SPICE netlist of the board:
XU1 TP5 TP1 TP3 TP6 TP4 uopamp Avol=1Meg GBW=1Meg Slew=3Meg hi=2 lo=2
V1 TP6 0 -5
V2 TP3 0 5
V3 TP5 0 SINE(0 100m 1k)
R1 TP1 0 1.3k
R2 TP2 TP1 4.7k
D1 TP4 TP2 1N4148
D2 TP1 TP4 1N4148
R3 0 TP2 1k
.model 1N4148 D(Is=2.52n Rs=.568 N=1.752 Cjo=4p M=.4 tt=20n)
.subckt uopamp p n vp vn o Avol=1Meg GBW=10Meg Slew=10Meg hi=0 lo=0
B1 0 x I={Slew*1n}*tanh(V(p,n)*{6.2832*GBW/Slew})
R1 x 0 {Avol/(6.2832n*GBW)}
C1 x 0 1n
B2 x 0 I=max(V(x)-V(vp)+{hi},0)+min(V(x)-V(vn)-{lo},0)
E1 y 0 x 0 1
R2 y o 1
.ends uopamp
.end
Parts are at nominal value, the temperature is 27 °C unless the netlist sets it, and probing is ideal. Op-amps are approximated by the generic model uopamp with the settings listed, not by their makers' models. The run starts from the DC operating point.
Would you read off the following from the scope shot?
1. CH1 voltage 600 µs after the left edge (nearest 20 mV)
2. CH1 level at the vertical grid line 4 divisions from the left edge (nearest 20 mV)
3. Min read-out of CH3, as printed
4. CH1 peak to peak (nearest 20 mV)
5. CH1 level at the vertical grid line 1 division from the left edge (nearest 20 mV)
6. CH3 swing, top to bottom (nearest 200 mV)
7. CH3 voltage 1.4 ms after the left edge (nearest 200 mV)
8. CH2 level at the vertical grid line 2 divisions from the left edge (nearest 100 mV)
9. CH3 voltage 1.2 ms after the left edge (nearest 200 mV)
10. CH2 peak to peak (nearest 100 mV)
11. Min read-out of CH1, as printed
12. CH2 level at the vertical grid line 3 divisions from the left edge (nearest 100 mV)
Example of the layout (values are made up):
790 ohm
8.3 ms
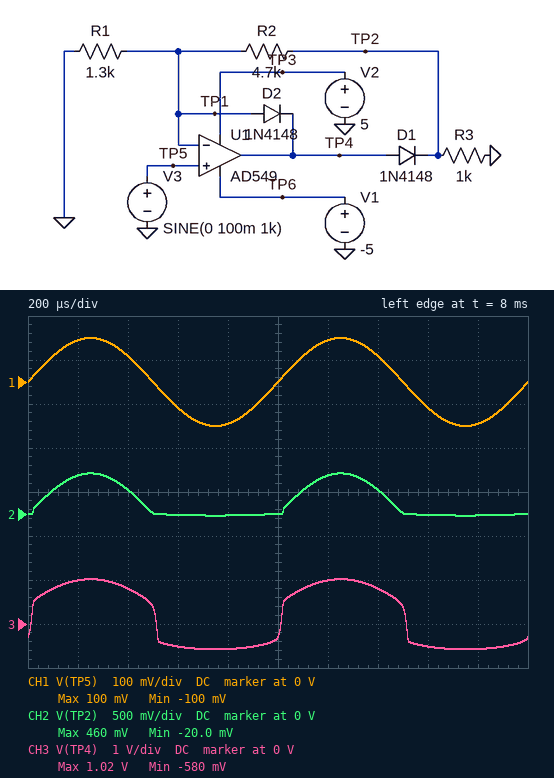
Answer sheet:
-60 mV
-100 mV
-580 mV
200 mV
100 mV
1.6 V
800 mV
300 mV
1.0 V
500 mV
-100 mV
0 V
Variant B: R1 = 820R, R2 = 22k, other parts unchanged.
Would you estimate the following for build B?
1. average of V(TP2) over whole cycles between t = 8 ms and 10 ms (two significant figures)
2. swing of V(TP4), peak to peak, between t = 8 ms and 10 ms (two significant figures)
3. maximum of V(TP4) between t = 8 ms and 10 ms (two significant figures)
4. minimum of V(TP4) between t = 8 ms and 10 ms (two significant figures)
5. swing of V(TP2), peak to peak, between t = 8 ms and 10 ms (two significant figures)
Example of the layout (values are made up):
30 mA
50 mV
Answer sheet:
830 mV
3.6 V
3.0 V
-590 mV
2.4 V
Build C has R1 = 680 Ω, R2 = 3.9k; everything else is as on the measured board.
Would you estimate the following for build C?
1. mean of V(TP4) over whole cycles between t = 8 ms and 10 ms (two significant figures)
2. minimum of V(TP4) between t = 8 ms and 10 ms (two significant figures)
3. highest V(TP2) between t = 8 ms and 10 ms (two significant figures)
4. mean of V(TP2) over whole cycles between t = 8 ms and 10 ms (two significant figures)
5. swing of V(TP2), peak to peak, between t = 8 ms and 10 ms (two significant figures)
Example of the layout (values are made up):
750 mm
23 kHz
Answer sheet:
220 mV
-600 mV
670 mV
210 mV
690 mV
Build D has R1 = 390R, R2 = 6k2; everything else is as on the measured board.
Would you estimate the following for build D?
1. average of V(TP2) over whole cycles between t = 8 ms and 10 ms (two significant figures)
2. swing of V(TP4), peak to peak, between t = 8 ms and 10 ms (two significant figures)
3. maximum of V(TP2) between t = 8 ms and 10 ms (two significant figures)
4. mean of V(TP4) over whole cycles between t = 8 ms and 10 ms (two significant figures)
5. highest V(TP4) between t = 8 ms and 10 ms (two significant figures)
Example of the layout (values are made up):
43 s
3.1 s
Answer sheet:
530 mV
2.9 V
1.7 V
550 mV
2.3 V
